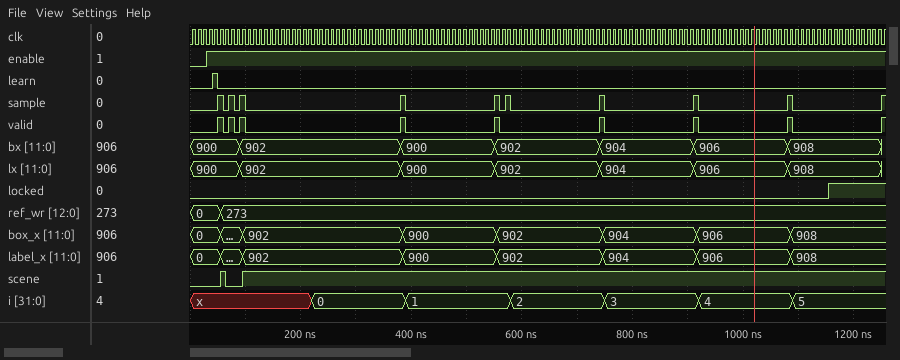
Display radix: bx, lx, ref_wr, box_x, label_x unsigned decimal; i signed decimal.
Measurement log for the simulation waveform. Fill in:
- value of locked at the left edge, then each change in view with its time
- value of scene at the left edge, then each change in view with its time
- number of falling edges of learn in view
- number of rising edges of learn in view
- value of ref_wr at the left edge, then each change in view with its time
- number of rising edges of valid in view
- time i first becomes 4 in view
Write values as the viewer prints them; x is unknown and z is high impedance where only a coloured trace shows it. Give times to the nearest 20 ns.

0, 1 at 1160 ns
0, 1 at 60 ns, 0 at 60 ns, 1 at 100 ns
1
1
0, 273 at 60 ns
9
920 ns
